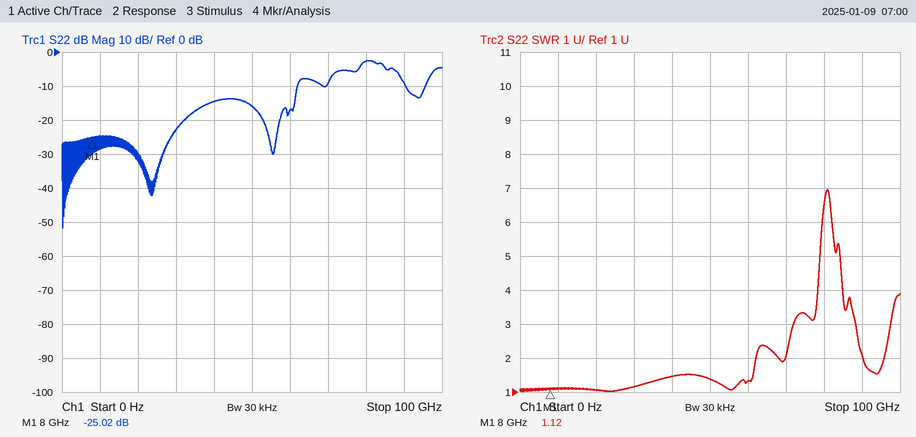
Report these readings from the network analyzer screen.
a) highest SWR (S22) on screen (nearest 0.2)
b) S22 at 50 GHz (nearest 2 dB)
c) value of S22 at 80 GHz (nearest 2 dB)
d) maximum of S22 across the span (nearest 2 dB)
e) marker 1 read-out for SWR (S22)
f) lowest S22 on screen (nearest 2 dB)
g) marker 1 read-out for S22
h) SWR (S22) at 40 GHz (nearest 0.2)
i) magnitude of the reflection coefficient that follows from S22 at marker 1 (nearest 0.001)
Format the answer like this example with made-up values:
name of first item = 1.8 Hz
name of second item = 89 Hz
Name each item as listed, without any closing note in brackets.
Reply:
highest SWR (S22) on screen = 7.0
S22 at 50 GHz = -16 dB
value of S22 at 80 GHz = -2 dB
maximum of S22 across the span = -2 dB
marker 1 read-out for SWR = 1.12
lowest S22 on screen = -52 dB
marker 1 read-out for S22 = -25.02 dB
SWR (S22) at 40 GHz = 1.4
magnitude of the reflection coefficient that follows from S22 at marker 1 = 0.056
